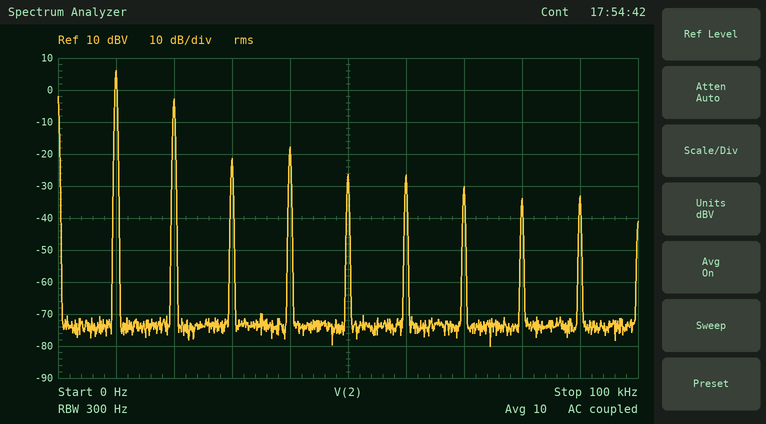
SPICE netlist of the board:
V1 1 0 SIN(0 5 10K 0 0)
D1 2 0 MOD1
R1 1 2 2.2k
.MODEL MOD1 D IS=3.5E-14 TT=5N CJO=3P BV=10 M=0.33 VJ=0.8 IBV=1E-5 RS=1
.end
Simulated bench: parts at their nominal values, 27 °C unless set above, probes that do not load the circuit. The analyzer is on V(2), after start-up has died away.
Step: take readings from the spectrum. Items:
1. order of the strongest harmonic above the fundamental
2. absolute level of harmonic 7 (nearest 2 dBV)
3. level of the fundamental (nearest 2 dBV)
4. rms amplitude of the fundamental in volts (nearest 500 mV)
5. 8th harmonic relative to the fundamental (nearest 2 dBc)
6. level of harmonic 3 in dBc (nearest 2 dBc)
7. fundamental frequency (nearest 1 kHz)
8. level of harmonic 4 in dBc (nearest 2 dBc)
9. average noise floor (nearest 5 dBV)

2
-30 dBV
6 dBV
2.0 V
-40 dBc
-28 dBc
10 kHz
-24 dBc
-75 dBV
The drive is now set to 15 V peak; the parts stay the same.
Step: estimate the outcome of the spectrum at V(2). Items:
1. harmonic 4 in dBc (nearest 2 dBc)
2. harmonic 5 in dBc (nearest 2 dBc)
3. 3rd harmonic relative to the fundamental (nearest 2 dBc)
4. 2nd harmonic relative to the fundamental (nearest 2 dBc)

-16 dBc
-46 dBc
-16 dBc
-10 dBc
